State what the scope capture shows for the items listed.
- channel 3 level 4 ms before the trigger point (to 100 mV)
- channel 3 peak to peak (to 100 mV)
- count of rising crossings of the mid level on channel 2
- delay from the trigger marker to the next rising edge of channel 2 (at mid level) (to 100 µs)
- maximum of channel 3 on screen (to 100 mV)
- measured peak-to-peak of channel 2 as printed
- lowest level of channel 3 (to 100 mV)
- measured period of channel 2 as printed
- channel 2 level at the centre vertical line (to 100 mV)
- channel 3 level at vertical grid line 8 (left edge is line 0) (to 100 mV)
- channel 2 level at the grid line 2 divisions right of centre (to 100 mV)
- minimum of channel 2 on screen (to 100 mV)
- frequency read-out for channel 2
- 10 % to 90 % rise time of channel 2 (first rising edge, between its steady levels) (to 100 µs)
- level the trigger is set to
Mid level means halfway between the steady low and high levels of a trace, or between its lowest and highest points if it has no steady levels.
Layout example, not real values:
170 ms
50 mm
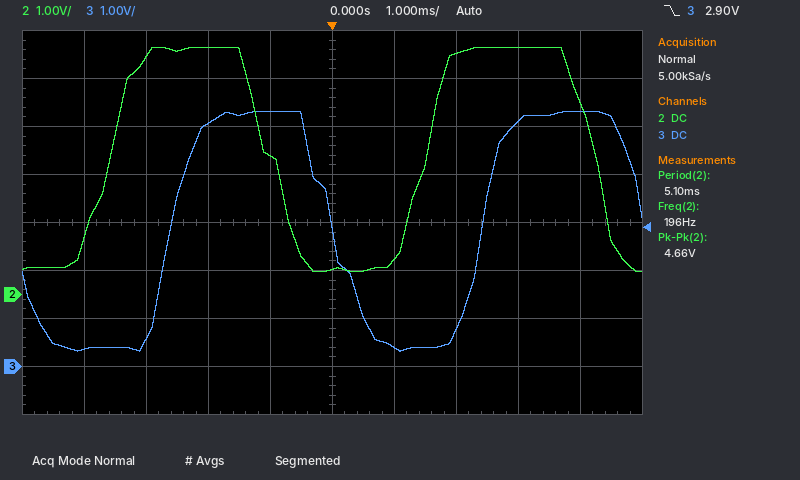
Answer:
400 mV
5.0 V
2
1.5 ms
5.3 V
4.66 V
300 mV
5.10 ms
500 mV
5.1 V
5.0 V
500 mV
196 Hz
900 µs
2.90 V
